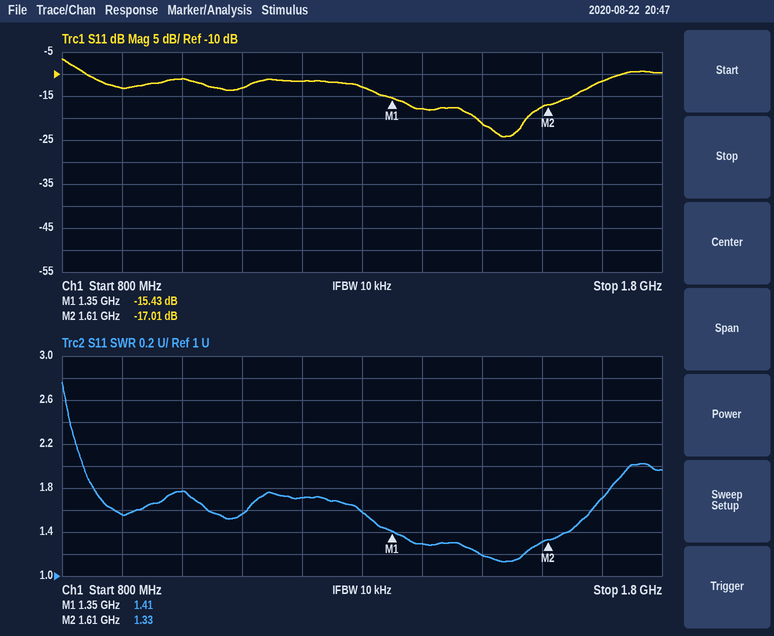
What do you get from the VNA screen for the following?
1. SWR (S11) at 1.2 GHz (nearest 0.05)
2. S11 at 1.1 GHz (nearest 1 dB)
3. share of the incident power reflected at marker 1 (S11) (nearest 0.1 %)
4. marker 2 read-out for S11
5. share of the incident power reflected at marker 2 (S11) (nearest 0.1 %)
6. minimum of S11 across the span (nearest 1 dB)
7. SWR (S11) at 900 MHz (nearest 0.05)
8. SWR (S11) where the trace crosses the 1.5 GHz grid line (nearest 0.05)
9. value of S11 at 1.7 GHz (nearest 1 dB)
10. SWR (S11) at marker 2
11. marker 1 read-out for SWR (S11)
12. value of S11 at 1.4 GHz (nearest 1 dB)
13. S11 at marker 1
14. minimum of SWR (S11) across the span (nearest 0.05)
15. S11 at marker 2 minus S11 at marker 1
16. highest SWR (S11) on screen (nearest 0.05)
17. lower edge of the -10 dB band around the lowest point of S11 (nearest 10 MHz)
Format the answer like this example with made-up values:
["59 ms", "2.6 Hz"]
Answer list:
["1.70", "-13 dB", "2.9 %", "-17.01 dB", "2.0 %", "-24 dB", "1.55", "1.20", "-12 dB", "1.33", "1.41", "-18 dB", "-15.43 dB", "1.15", "-1.58 dB", "2.75", "840 MHz"]
